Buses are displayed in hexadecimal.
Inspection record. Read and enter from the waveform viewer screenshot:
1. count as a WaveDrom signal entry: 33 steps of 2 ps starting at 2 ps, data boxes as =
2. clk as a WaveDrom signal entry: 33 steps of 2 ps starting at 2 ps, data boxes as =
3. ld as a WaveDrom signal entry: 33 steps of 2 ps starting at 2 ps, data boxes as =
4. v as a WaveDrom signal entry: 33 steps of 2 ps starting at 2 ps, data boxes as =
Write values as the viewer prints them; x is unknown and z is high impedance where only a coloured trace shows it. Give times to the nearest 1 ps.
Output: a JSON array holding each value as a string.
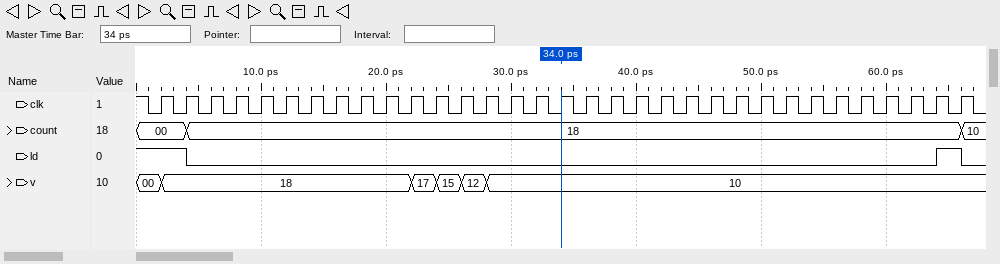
["{name: 'count', wave: '==..............................=', data: '00 18 10'}", "{name: 'clk', wave: 'p................................'}", "{name: 'ld', wave: '10.............................10'}", "{name: 'v', wave: '=.........====...................', data: '18 17 15 12 10'}"]
